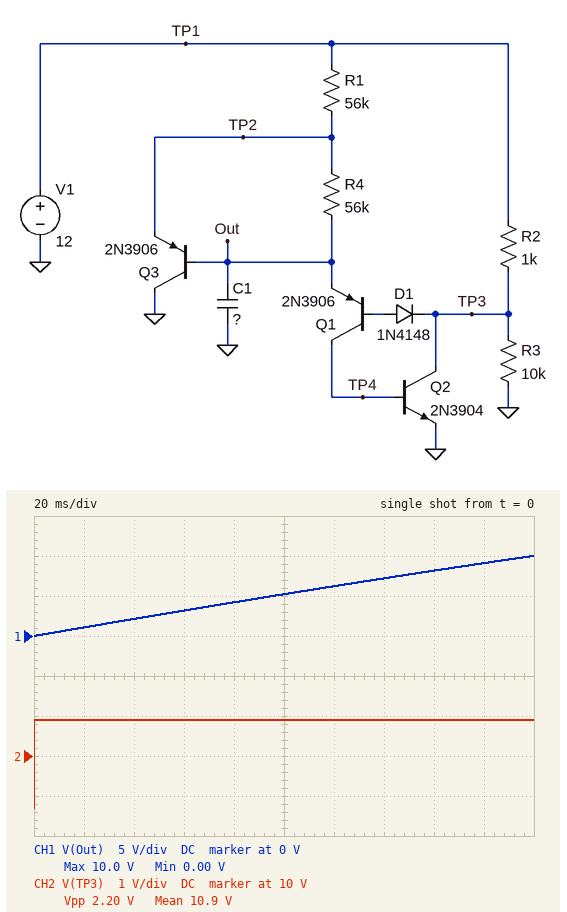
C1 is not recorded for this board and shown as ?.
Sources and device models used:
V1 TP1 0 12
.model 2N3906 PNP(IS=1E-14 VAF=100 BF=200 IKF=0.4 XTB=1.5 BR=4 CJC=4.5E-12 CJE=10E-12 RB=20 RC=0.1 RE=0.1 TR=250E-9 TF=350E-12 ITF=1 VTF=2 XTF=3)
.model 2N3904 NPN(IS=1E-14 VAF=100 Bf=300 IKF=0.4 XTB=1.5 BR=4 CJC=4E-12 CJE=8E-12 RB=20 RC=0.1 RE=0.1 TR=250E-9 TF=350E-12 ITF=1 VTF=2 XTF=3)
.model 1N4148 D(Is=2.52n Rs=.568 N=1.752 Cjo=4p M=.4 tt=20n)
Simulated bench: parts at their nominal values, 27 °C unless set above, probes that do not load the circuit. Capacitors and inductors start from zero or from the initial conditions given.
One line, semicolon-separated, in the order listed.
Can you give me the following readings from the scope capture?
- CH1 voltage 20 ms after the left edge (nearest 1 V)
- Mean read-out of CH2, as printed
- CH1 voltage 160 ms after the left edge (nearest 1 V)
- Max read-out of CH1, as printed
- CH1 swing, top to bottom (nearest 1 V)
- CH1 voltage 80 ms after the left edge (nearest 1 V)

1 V; 10.9 V; 8 V; 10.0 V; 10 V; 4 V
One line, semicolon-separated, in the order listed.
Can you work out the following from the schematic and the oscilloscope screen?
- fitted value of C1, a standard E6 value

220 nF
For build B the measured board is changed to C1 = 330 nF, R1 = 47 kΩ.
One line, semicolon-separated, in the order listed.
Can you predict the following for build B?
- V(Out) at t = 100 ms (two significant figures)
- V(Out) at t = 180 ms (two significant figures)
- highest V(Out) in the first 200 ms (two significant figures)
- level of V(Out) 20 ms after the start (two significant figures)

3.6 V; 6.3 V; 7.0 V; 730 mV
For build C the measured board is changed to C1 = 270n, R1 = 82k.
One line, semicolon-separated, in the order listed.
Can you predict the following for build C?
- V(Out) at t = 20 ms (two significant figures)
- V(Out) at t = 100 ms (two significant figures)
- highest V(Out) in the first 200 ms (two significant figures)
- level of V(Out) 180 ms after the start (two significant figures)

840 mV; 4.1 V; 8.0 V; 7.3 V
